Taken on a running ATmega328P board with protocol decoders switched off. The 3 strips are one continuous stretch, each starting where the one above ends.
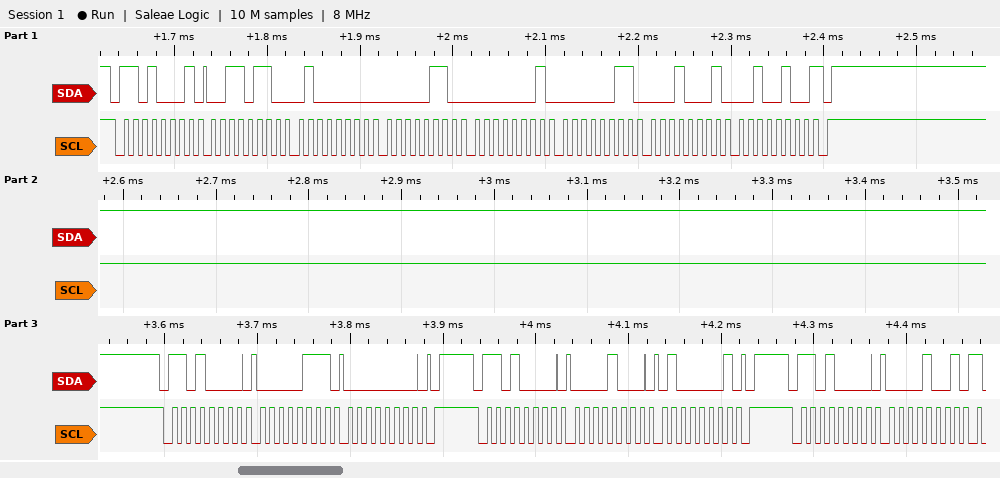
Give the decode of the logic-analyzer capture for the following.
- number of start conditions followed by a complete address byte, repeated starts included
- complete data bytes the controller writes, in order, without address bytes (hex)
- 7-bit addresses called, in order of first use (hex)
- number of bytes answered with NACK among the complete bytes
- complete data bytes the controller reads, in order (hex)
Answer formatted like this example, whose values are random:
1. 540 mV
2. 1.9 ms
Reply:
1. 4
2. 07 00 08 41 09
3. 0x68
4. 1
5. 36 40 06 01 03 11 24
